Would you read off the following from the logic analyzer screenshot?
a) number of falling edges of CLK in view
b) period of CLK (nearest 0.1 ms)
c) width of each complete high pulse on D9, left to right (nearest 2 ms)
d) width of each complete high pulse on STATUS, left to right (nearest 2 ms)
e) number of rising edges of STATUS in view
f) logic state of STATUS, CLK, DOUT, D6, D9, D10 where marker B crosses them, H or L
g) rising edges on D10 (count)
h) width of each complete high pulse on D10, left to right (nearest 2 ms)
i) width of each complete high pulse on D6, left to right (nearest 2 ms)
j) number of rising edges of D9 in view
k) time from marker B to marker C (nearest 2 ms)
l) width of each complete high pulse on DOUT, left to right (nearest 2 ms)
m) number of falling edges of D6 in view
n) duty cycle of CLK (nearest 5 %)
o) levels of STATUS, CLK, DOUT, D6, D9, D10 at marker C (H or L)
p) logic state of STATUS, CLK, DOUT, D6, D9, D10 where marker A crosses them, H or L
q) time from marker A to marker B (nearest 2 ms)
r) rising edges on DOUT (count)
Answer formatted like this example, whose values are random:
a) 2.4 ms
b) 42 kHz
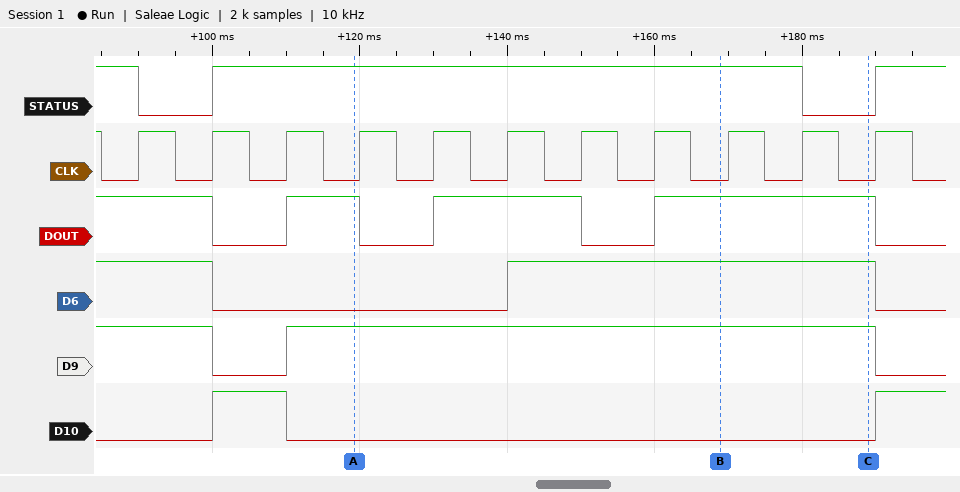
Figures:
a) 12
b) 10 ms
c) 80 ms
d) 80 ms
e) 2
f) STATUS=H, CLK=L, DOUT=H, D6=H, D9=H, D10=L
g) 2
h) 10 ms
i) 50 ms
j) 1
k) 20 ms
l) 10 ms, 20 ms, 30 ms
m) 2
n) 50 %
o) STATUS=L, CLK=L, DOUT=H, D6=H, D9=H, D10=L
p) STATUS=H, CLK=L, DOUT=H, D6=L, D9=H, D10=L
q) 50 ms
r) 3
